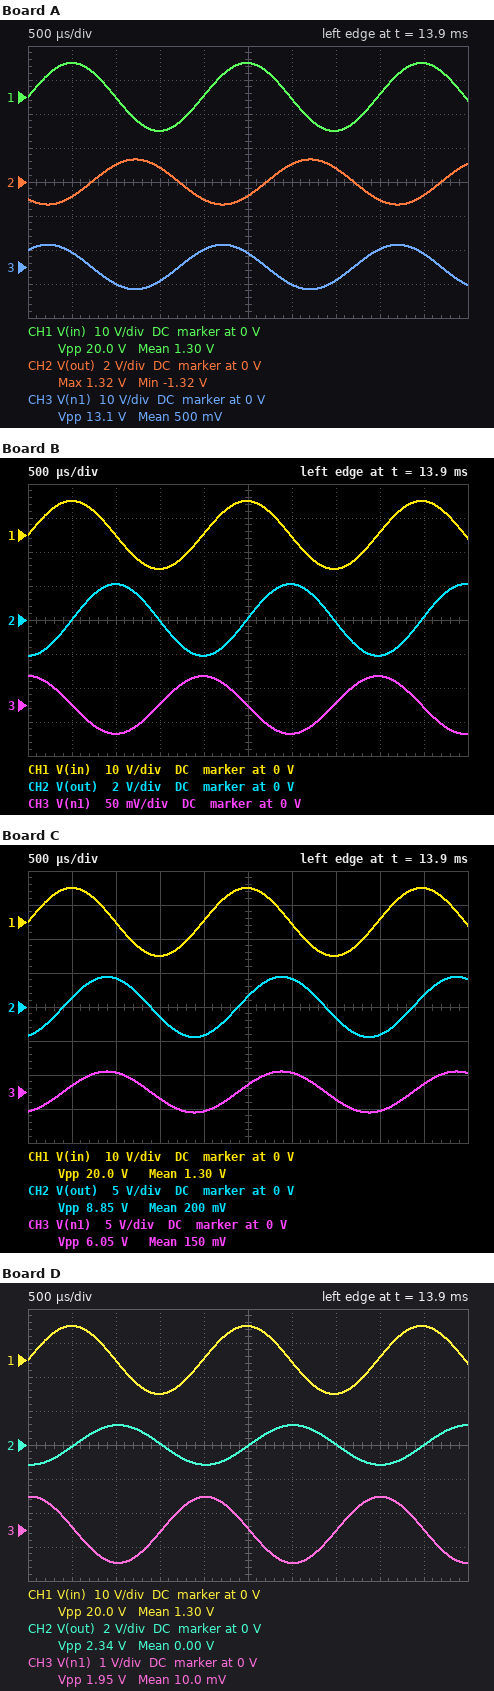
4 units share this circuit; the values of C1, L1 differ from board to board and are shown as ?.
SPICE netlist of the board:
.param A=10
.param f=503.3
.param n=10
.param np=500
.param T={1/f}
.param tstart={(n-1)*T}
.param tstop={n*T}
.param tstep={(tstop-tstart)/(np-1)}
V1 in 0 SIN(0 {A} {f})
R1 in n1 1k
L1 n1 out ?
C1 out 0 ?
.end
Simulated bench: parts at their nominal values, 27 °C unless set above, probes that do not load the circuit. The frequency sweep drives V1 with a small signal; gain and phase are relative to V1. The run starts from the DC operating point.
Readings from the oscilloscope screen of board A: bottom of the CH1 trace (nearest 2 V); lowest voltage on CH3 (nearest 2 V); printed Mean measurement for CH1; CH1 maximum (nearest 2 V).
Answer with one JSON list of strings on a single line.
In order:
["-10 V", "-6 V", "1.30 V", "10 V"]
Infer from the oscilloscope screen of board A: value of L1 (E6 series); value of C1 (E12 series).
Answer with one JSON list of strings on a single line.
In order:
["330 mH", "1.8 µF"]
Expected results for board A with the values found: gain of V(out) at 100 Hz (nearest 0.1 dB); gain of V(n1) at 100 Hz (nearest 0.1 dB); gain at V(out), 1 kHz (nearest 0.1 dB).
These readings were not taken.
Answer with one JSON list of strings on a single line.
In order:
["-2.7 dB", "-5.0 dB", "-28.0 dB"]
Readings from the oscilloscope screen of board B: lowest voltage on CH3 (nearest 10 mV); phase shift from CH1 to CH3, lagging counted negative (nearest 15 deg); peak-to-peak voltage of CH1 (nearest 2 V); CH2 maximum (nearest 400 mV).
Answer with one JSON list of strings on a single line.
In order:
["-40 mV", "90 deg", "20 V", "2.0 V"]
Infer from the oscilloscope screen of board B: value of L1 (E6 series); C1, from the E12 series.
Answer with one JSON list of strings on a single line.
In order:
["68 mH", "1.5 µF"]
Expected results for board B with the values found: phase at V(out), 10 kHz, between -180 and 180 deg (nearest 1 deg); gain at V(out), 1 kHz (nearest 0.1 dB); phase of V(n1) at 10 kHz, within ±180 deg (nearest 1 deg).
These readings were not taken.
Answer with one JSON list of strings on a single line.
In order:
["-167 deg", "-19.9 dB", "13 deg"]
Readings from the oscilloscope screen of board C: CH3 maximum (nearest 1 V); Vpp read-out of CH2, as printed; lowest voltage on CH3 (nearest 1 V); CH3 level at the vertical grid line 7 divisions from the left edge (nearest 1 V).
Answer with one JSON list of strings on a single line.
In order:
["3 V", "8.85 V", "-3 V", "-1 V"]
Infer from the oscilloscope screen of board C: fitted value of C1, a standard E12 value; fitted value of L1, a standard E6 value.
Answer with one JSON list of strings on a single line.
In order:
["680 nF", "47 mH"]
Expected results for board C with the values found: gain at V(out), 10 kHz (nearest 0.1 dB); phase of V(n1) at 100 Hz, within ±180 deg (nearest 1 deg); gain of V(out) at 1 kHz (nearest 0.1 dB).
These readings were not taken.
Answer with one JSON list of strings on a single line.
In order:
["-42.4 dB", "-23 deg", "-12.6 dB"]
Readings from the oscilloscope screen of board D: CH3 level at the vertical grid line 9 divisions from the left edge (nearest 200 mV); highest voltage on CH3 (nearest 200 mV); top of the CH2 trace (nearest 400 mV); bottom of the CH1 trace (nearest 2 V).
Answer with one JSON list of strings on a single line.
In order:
["0 V", "1.0 V", "1.2 V", "-10 V"]
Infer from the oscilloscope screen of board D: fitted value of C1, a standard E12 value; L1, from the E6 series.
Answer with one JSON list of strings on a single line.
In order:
["2.7 µF", "68 mH"]
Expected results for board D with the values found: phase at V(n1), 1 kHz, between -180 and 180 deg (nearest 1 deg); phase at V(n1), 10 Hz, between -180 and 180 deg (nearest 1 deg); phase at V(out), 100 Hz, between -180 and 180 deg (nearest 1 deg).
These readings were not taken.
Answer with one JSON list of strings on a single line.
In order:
["70 deg", "-10 deg", "-61 deg"]
